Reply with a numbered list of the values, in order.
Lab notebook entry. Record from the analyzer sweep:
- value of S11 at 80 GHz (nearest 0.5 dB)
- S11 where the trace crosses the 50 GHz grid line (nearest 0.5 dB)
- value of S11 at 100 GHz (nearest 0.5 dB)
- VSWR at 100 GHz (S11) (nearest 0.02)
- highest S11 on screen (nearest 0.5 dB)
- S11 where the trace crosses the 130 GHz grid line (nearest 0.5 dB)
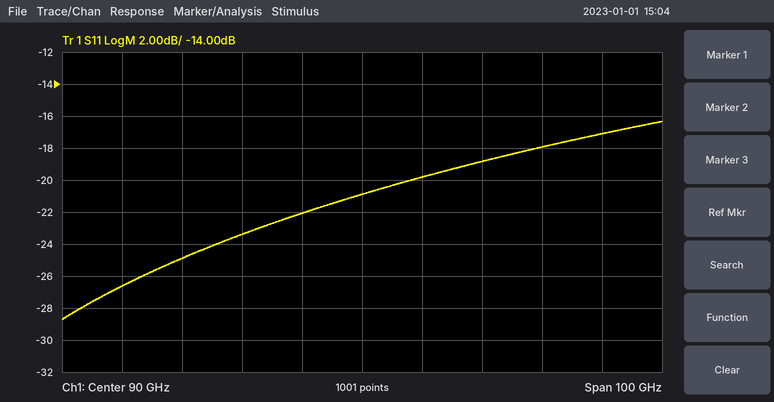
1. -22.0 dB
2. -26.5 dB
3. -20.0 dB
4. 1.22
5. -16.5 dB
6. -17.0 dB
